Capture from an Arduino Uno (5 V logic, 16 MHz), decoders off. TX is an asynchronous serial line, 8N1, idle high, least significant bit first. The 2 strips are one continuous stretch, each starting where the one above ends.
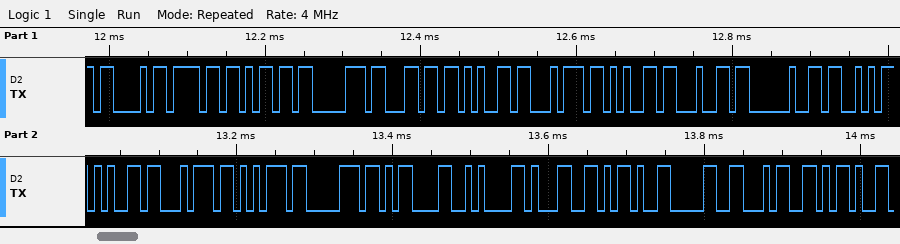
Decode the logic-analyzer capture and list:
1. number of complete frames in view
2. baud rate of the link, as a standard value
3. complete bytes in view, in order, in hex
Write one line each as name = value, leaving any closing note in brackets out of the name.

number of complete frames in view = 22
baud rate of the link, as a standard value = 115200 baud
complete bytes in view, in order, in hex = 43 6F 6D 70 6C 65 74 65 64 20 53 65 74 75 70 0D 0A 31 2D 30 34 2D
